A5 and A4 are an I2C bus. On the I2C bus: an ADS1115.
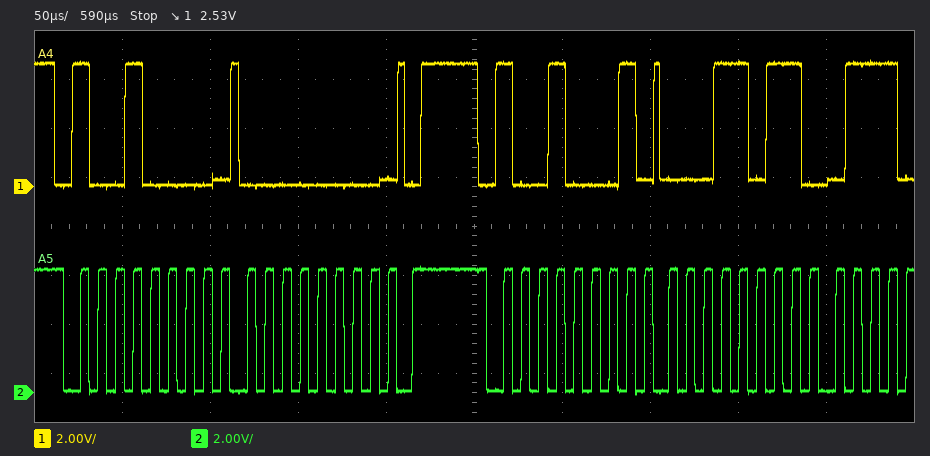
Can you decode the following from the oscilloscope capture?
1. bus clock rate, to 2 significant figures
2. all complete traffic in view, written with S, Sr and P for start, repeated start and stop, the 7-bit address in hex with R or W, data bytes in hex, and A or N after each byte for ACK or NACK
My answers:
100 kHz
S 48W A 00 A P S 48R A 1B A
